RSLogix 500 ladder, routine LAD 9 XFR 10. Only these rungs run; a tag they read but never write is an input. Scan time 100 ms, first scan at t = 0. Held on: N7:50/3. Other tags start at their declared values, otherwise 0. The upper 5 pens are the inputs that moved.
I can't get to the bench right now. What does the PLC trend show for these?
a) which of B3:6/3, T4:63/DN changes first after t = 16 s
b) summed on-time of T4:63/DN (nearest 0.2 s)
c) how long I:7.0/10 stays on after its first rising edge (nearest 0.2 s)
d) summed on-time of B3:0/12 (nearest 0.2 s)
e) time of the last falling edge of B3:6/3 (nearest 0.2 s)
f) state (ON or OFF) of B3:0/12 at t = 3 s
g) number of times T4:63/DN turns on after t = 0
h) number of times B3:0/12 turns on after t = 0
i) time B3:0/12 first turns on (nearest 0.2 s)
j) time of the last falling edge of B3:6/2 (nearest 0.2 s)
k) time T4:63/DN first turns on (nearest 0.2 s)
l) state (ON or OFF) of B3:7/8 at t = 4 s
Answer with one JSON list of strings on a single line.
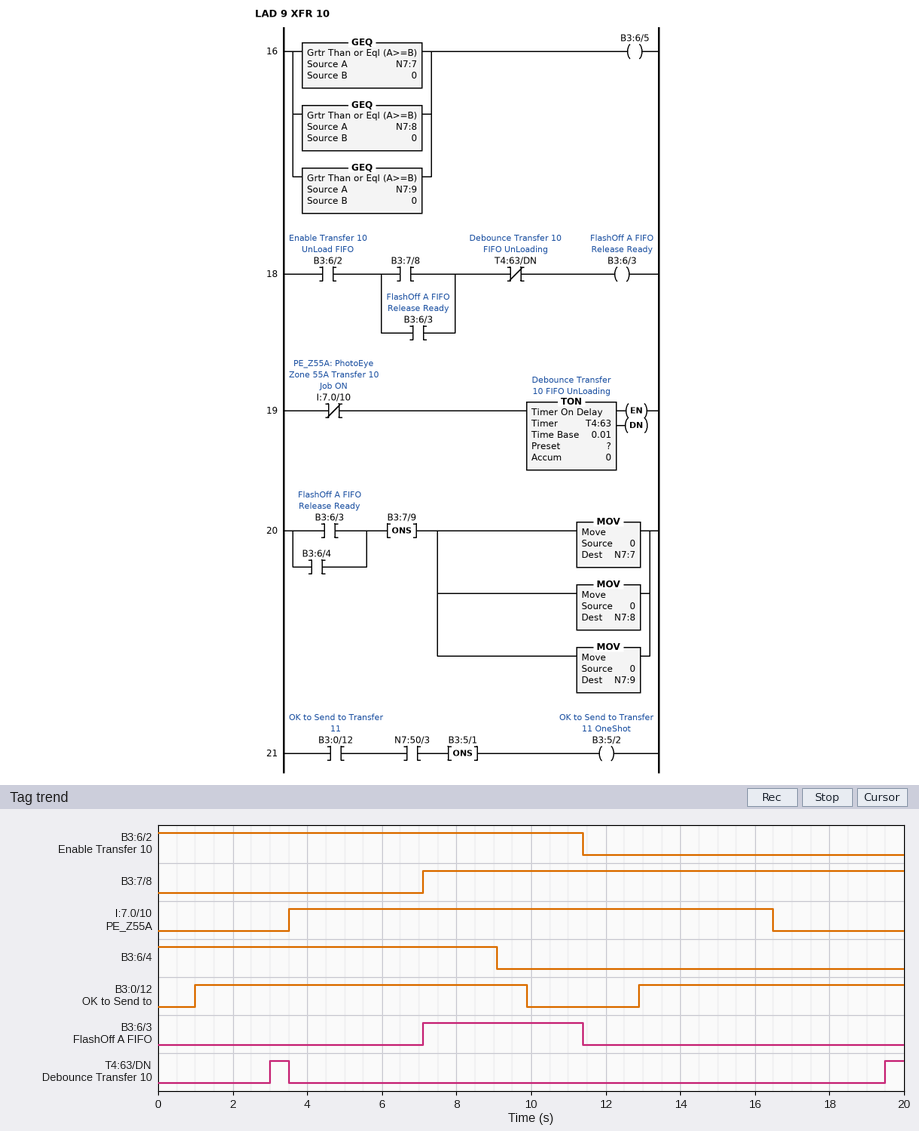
["T4:63/DN", "1.0 s", "13.0 s", "16.0 s", "11.4 s", "ON", "2", "2", "1.0 s", "11.4 s", "3.0 s", "OFF"]
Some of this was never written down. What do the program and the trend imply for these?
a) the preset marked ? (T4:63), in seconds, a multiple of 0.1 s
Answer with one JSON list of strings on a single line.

["3.0 s"]
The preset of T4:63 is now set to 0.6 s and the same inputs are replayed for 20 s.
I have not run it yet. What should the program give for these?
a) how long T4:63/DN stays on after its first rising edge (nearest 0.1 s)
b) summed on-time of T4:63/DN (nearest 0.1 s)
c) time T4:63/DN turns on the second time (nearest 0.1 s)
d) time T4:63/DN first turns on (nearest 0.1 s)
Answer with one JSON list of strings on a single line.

["2.9 s", "5.8 s", "17.1 s", "0.6 s"]
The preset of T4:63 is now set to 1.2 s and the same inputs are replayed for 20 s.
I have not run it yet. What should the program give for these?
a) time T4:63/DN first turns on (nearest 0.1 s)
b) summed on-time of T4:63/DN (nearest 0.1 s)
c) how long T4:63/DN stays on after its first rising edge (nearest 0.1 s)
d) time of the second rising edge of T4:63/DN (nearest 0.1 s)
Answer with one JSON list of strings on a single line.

["1.2 s", "4.6 s", "2.3 s", "17.7 s"]
